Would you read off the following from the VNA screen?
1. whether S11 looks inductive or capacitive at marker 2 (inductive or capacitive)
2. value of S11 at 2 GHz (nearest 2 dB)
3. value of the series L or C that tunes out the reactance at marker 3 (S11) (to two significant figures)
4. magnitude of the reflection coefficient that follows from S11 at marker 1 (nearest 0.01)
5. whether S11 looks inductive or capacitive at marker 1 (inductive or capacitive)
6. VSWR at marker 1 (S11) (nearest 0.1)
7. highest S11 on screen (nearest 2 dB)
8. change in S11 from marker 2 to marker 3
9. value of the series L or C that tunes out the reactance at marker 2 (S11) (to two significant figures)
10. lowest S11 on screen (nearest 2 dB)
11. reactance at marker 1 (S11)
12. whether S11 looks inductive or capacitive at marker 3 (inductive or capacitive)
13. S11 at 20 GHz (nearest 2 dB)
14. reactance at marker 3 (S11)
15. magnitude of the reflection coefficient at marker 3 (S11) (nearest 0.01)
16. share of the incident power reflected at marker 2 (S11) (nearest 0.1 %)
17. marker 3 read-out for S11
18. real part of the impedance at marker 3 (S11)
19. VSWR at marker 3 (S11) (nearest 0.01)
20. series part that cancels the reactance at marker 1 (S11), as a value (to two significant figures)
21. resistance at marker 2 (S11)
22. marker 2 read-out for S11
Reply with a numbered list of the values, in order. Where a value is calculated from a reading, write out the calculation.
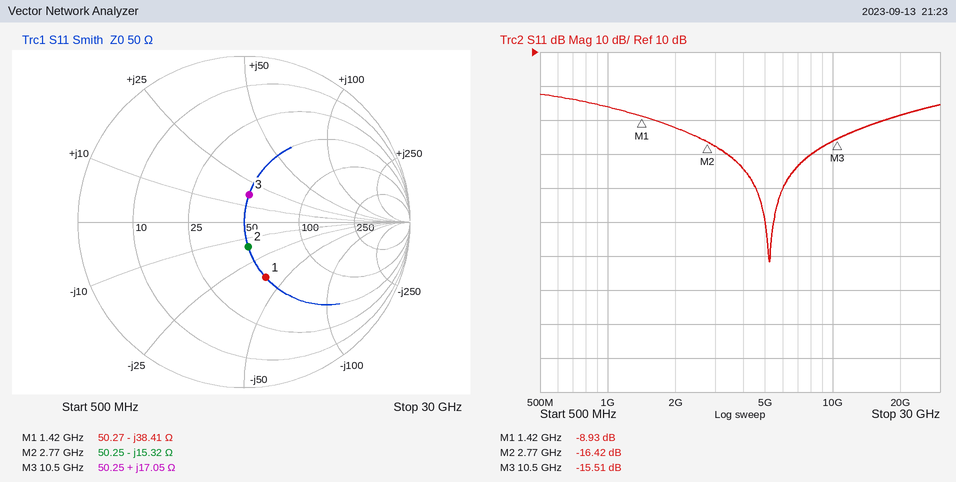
1. capacitive
2. -12 dB
3. C = 1/(2π × 10.5 GHz × 17.05 Ω) ≈ 889 fF, so 890 fF to two significant figures
4. 10^(-8.93/20) ≈ 0.36
5. capacitive
6. 2.1
7. -2 dB
8. -15.51 − (-16.42) = 0.91 dB
9. L = 15.32 Ω/(2π × 2.77 GHz) ≈ 880 pH
10. -52 dB
11. -38.41 Ω
12. inductive
13. -8 dB
14. +17.05 Ω
15. 10^(-15.51/20) ≈ 0.17
16. 10^(-16.42/10) ≈ 2.3 %
17. -15.51 dB
18. 50.25 Ω
19. 1.40
20. L = 38.41 Ω/(2π × 1.42 GHz) ≈ 4.3 nH
21. 50.25 Ω
22. -16.42 dB
